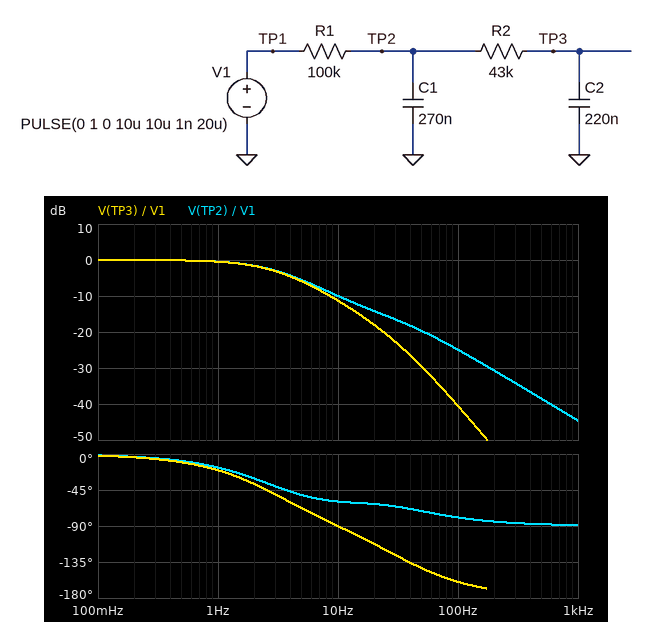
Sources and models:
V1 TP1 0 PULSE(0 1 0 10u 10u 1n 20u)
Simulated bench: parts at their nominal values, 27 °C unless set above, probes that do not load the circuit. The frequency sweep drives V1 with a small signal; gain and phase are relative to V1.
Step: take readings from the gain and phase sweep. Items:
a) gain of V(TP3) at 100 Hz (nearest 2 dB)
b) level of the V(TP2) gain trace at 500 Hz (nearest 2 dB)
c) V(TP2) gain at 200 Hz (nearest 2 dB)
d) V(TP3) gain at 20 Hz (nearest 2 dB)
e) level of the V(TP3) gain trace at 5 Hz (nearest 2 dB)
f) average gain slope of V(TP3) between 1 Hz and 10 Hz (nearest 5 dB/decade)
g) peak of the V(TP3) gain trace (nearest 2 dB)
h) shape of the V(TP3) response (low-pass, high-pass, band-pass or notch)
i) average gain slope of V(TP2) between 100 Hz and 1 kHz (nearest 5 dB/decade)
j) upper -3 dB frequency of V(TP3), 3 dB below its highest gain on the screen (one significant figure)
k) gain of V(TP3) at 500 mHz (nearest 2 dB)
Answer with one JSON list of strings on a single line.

["-40 dB", "-38 dB", "-30 dB", "-18 dB", "-6 dB", "-10 dB/decade", "0 dB", "low-pass", "-20 dB/decade", "3 Hz", "0 dB"]
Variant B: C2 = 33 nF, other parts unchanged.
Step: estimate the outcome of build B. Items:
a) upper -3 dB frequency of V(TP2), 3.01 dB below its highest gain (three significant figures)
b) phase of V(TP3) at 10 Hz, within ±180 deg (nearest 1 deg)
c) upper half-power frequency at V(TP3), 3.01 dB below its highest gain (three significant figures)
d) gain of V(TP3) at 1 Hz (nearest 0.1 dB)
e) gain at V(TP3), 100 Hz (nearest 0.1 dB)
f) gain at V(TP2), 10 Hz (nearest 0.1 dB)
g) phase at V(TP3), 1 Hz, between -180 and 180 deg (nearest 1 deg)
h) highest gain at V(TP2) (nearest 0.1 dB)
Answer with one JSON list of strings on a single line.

["5.23 Hz", "-67 deg", "5.22 Hz", "-0.2 dB", "-27.8 dB", "-6.7 dB", "-11 deg", "0 dB"]
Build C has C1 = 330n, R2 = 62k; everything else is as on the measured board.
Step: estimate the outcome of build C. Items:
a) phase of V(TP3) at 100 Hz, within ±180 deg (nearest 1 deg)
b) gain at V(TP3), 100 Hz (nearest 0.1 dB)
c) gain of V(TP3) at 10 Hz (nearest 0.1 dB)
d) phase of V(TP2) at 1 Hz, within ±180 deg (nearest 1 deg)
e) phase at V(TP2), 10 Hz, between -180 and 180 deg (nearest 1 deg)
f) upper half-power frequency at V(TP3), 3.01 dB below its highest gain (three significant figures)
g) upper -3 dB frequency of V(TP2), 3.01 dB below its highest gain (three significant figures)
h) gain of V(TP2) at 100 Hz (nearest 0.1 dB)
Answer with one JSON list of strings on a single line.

["-166 deg", "-45.2 dB", "-12.8 dB", "-19 deg", "-60 deg", "2.56 Hz", "2.69 Hz", "-26.5 dB"]
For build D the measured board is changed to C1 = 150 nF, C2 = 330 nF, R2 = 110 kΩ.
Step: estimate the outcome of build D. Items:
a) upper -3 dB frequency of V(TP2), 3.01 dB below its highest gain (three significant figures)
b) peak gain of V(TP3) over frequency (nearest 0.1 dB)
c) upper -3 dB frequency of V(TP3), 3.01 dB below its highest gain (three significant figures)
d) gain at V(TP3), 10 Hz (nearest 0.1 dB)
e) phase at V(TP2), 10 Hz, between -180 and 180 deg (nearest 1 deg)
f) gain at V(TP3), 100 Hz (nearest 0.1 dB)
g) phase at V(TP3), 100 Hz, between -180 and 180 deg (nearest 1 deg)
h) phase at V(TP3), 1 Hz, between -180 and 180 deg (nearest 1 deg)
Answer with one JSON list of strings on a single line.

["2.70 Hz", "0 dB", "2.04 Hz", "-14.7 dB", "-36 deg", "-46.9 dB", "-166 deg", "-28 deg"]
